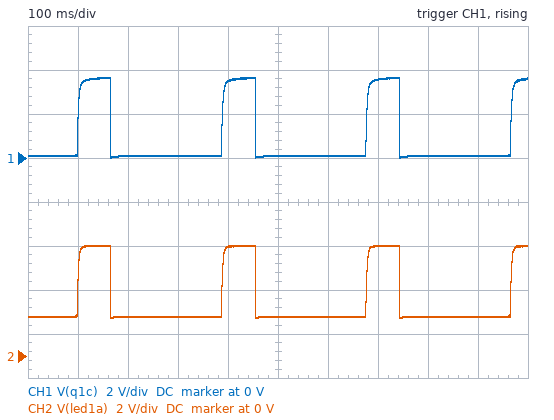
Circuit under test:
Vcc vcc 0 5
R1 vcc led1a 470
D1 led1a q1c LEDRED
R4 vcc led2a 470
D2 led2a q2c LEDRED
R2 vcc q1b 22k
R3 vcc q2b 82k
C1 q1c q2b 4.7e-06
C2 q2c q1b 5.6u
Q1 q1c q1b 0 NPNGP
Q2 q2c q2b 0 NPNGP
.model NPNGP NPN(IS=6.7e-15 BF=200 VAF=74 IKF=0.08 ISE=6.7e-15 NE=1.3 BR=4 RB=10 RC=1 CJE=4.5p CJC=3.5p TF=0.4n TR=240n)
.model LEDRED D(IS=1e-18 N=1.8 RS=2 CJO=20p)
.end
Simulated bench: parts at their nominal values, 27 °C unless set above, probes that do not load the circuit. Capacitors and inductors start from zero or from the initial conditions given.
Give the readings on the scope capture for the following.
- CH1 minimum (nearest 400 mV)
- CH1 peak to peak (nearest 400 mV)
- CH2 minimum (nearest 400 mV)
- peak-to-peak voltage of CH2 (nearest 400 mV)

0 V
3.6 V
1.6 V
3.2 V
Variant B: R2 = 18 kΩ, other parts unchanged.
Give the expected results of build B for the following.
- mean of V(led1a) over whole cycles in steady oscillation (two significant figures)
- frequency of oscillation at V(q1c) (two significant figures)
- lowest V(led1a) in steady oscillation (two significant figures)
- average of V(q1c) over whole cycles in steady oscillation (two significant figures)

2.4 V
3.6 Hz
1.7 V
740 mV
